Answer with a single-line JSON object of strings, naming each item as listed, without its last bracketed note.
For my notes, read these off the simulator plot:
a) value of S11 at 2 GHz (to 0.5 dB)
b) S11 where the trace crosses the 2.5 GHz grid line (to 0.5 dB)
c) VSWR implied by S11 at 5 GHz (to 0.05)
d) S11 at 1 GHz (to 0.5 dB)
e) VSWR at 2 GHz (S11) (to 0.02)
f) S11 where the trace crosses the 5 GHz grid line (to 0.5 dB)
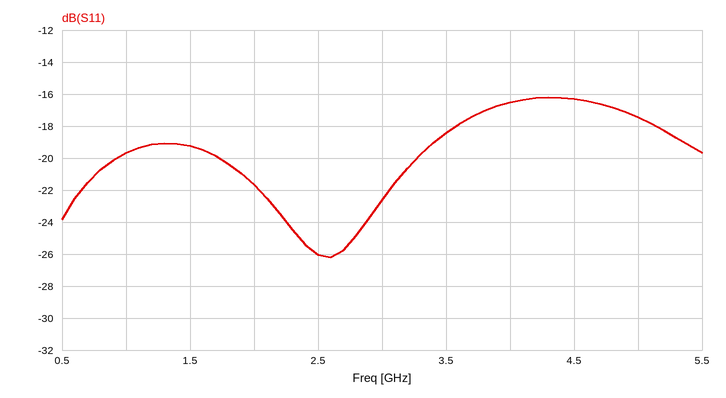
{"value of S11 at 2 GHz": "-21.5 dB", "S11 where the trace crosses the 2.5 GHz grid line": "-26.0 dB", "VSWR implied by S11 at 5 GHz": "1.30", "S11 at 1 GHz": "-19.5 dB", "VSWR at 2 GHz (S11)": "1.18", "S11 where the trace crosses the 5 GHz grid line": "-17.5 dB"}
